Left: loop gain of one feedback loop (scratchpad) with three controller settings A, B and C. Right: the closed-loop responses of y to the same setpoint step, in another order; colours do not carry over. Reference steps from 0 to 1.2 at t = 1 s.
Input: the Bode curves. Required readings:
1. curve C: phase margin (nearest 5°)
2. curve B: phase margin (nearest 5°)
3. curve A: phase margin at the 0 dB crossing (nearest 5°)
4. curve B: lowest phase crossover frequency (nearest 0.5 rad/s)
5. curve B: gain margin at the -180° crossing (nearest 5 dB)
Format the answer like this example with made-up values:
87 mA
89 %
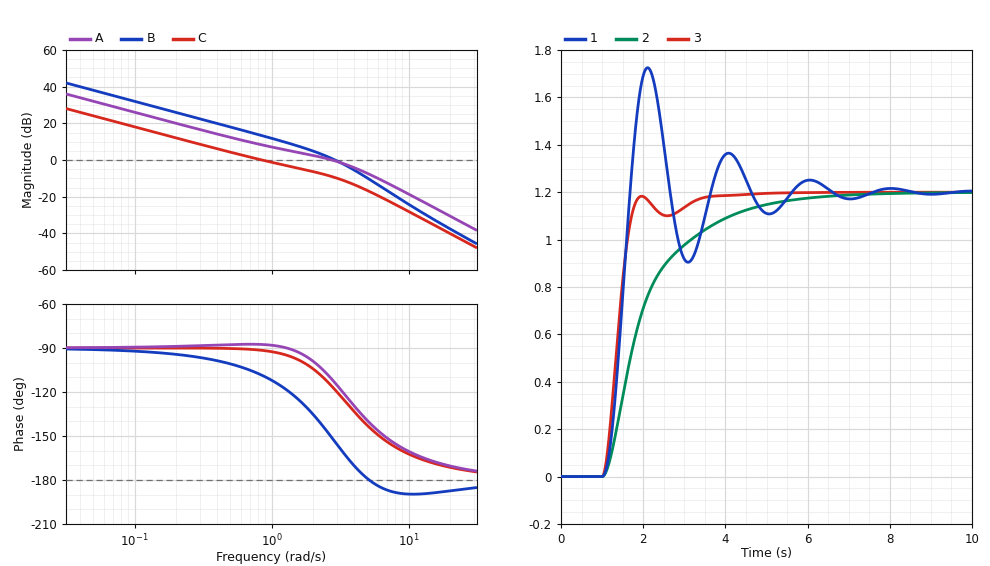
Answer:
90°
25°
70°
5.0 rad/s
10 dB
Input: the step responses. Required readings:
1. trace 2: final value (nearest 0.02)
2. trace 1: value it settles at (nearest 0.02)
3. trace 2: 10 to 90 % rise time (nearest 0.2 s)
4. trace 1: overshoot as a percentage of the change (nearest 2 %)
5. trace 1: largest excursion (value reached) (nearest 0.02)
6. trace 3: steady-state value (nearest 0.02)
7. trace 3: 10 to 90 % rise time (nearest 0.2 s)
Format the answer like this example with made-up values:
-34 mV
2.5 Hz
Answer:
1.20
1.20
2.6 s
44 %
1.72
1.20
0.6 s
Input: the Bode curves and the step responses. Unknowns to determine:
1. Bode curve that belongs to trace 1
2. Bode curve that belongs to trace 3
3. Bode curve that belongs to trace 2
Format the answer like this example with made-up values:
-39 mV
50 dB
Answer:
B
A
C
